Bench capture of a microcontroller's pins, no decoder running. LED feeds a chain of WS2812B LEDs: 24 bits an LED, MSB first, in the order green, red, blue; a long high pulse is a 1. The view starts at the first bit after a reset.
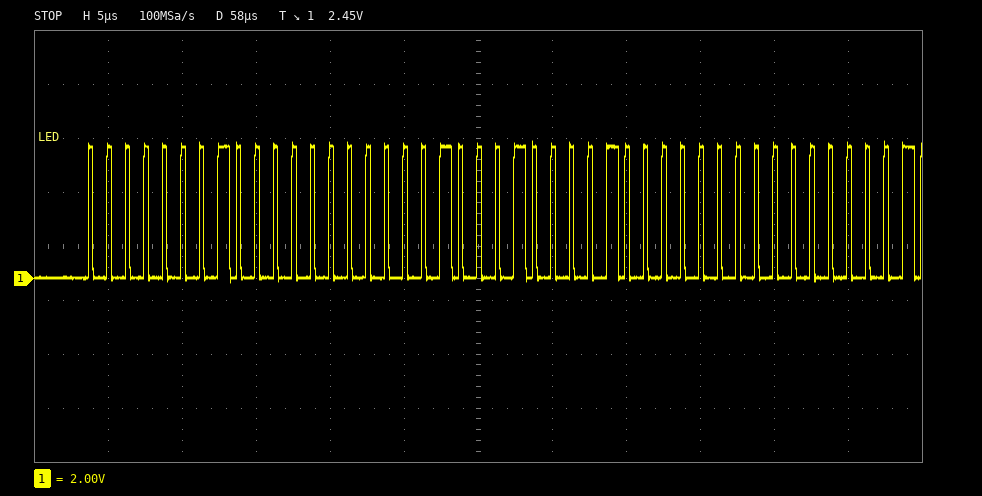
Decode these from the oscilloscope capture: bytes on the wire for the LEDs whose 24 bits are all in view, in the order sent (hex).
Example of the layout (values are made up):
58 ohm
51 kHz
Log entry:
01 00 11
